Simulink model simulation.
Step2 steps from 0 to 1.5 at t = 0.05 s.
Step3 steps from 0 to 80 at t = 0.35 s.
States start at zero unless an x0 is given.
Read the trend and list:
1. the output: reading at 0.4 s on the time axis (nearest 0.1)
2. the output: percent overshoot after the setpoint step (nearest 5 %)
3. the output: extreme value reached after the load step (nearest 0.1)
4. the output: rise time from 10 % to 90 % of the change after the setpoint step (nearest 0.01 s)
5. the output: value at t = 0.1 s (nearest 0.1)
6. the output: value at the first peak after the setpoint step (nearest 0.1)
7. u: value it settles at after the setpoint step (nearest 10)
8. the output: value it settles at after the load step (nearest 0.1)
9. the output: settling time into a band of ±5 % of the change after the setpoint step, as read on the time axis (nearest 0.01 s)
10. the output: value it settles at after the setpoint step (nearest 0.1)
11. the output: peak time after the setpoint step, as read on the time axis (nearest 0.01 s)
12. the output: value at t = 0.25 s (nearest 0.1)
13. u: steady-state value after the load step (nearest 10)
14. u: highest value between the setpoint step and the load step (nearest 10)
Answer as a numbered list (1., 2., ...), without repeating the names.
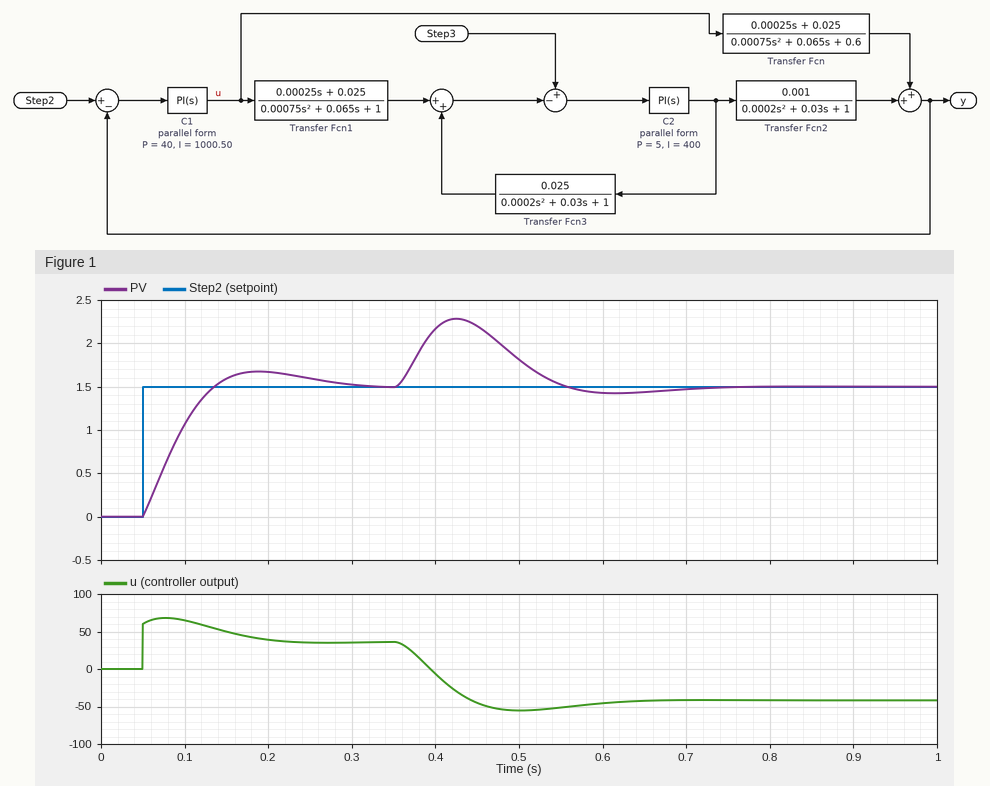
1. 2.2
2. 10 %
3. 2.3
4. 0.06 s
5. 1.1
6. 1.7
7. 40
8. 1.5
9. 0.26 s
10. 1.5
11. 0.19 s
12. 1.6
13. -40
14. 70
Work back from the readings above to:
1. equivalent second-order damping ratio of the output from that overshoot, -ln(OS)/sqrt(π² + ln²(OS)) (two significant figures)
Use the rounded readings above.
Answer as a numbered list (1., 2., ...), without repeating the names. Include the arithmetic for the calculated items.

1. ln(0.1) = -2.303; 2.303 / sqrt(9.870 + 5.302) = 0.59
